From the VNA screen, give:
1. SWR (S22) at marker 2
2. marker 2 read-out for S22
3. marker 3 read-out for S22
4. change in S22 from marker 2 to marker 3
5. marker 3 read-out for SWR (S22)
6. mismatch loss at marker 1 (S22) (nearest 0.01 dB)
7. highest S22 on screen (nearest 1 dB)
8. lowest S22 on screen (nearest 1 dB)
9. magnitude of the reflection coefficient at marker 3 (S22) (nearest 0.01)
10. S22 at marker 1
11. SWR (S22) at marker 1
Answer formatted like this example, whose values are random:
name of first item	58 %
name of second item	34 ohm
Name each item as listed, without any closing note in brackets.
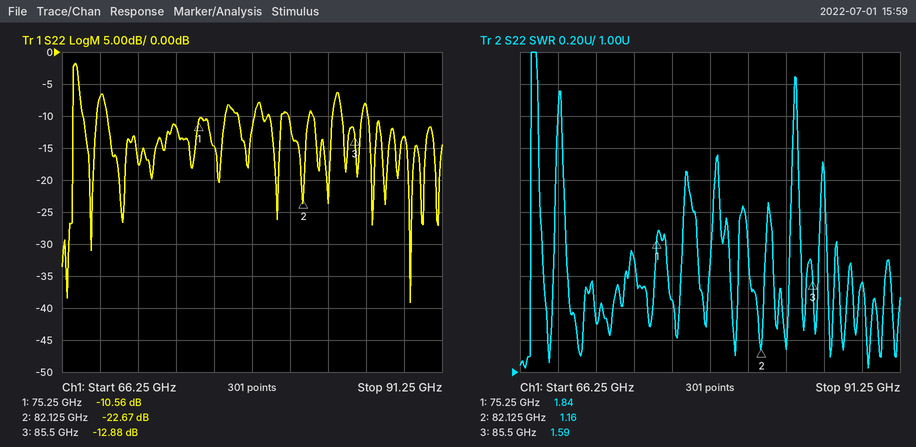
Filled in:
SWR (S22) at marker 2	1.16
marker 2 read-out for S22	-22.67 dB
marker 3 read-out for S22	-12.88 dB
change in S22 from marker 2 to marker 3	9.79 dB
marker 3 read-out for SWR	1.59
mismatch loss at marker 1 (S22)	0.40 dB
highest S22 on screen	-2 dB
lowest S22 on screen	-39 dB
magnitude of the reflection coefficient at marker 3 (S22)	0.23
S22 at marker 1	-10.56 dB
SWR (S22) at marker 1	1.84
